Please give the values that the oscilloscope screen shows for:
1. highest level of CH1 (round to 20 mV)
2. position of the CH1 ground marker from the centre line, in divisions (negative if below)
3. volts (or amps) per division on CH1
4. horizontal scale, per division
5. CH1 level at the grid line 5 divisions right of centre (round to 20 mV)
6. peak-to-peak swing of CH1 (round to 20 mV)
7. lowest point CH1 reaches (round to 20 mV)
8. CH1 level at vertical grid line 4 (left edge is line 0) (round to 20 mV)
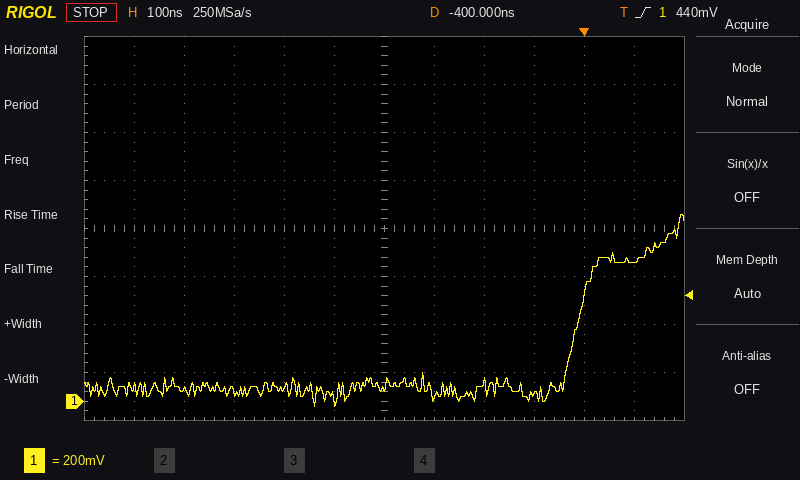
780 mV
-3.6 div
200 mV
100 ns
580 mV
800 mV
-20 mV
60 mV
